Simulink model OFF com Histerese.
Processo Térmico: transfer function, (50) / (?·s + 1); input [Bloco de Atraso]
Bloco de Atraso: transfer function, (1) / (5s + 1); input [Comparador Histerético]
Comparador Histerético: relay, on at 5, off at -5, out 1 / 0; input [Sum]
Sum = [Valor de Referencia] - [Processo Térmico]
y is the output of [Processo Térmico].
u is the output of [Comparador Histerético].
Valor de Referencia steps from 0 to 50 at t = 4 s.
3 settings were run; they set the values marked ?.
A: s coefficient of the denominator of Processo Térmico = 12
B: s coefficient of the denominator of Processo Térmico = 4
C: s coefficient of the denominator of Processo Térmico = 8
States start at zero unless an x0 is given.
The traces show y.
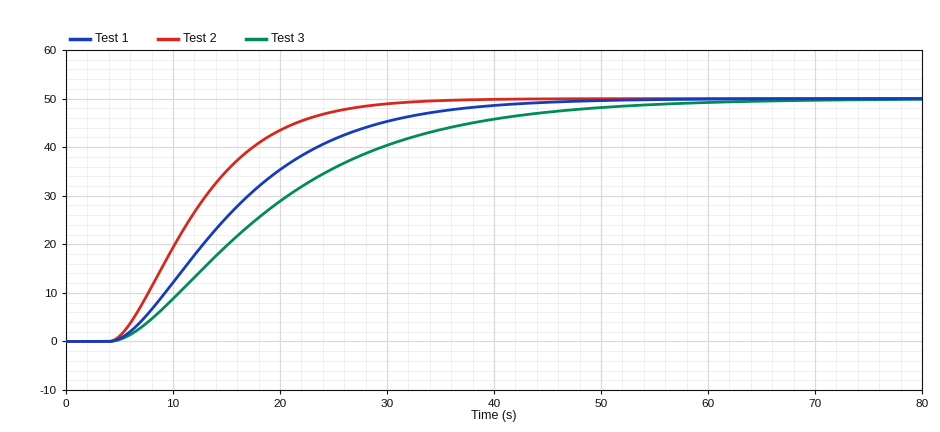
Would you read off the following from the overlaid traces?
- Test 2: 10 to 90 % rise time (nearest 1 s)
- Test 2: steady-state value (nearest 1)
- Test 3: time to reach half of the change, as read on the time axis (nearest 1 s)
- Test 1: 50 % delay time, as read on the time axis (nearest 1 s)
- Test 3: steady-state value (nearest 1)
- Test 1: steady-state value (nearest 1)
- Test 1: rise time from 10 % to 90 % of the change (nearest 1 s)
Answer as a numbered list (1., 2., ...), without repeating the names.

1. 15 s
2. 50
3. 18 s
4. 15 s
5. 50
6. 50
7. 22 s
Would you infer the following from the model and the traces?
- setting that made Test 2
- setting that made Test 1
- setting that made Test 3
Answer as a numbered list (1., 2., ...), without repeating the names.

1. B
2. C
3. A
